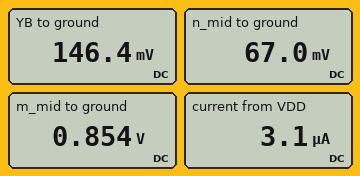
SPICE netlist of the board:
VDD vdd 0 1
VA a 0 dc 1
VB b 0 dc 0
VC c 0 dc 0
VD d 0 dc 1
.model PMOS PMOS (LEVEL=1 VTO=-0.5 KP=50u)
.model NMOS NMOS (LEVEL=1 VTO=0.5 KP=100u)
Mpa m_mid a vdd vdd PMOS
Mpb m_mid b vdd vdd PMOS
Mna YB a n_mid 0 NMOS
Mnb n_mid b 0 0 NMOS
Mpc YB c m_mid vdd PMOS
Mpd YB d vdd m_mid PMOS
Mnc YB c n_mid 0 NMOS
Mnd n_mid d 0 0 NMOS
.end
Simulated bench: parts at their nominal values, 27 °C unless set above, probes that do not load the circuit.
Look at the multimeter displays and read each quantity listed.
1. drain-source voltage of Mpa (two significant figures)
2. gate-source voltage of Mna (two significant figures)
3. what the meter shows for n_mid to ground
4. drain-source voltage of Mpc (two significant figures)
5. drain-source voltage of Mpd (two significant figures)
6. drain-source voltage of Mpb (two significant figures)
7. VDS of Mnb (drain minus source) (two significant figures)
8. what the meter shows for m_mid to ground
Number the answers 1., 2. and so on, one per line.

1. -150 mV
2. 930 mV
3. 67.0 mV
4. -710 mV
5. -850 mV
6. -150 mV
7. 67 mV
8. 0.854 V
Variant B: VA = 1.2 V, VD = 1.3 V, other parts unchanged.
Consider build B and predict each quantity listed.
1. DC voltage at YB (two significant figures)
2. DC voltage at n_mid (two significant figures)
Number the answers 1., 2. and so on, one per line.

1. 89 mV
2. 40 mV
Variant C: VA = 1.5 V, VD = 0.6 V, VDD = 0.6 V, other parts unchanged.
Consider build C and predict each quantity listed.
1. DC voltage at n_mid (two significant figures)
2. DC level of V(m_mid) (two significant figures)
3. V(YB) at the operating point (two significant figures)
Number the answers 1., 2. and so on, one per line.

1. 13 mV
2. 570 mV
3. 15 mV
